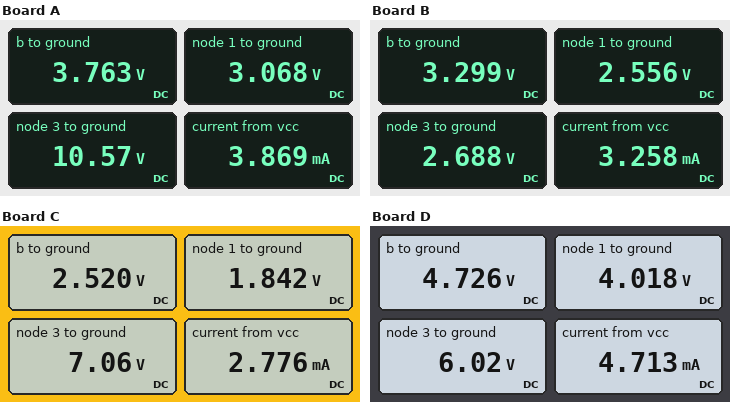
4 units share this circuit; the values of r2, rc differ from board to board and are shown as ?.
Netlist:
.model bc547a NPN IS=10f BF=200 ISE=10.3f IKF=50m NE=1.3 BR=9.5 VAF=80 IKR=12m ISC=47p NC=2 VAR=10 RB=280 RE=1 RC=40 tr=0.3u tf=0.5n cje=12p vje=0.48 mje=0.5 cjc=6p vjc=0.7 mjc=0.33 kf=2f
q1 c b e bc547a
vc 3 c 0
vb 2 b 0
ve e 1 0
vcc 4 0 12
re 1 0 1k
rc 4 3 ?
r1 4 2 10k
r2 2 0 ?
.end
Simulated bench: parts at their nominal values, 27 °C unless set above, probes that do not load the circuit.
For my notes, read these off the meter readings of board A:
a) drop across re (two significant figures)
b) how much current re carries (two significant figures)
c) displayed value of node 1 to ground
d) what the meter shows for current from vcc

3.1 V
3.1 mA
3.068 V
3.869 mA
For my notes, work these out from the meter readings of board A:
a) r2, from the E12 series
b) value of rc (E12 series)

4.7 kΩ
470 Ω
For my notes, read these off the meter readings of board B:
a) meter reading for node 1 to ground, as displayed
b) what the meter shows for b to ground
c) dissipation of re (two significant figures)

2.556 V
3.299 V
6.5 mW
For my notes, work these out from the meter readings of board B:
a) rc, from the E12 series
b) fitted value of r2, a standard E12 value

3.9 kΩ
4.7 kΩ
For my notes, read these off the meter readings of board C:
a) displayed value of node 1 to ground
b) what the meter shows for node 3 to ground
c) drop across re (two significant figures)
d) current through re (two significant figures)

1.842 V
7.06 V
1.8 V
1.8 mA
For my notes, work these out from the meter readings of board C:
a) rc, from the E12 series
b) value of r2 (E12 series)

2.7 kΩ
2.7 kΩ
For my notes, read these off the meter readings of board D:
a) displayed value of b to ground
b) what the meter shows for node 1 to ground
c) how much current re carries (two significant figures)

4.726 V
4.018 V
4.0 mA
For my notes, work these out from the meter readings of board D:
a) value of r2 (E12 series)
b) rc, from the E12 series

6.8 kΩ
1.5 kΩ
